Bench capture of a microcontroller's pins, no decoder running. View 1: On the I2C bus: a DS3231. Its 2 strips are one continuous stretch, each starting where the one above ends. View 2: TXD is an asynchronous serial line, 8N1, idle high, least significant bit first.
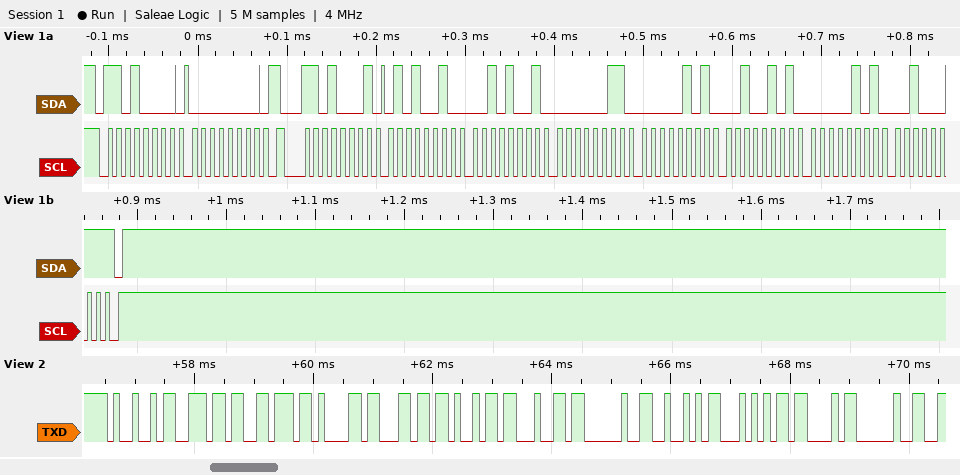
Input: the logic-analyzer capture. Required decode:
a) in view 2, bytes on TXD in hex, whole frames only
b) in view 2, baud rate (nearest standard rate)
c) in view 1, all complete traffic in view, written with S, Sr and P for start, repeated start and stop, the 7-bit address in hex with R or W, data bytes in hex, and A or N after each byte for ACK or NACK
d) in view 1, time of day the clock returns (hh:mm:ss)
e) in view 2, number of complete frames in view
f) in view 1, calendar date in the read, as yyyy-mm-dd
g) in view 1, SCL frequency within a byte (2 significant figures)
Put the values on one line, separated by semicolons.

49 6E 76 61 6C 69 64 20 52 54 43 20; 9600 baud; S 68W A 00 A Sr 68R A 52 A 29 A 03 A 05 A 25 A 05 A 23 N P; 03:29:52; 12; 2023-05-25; 100 kHz
